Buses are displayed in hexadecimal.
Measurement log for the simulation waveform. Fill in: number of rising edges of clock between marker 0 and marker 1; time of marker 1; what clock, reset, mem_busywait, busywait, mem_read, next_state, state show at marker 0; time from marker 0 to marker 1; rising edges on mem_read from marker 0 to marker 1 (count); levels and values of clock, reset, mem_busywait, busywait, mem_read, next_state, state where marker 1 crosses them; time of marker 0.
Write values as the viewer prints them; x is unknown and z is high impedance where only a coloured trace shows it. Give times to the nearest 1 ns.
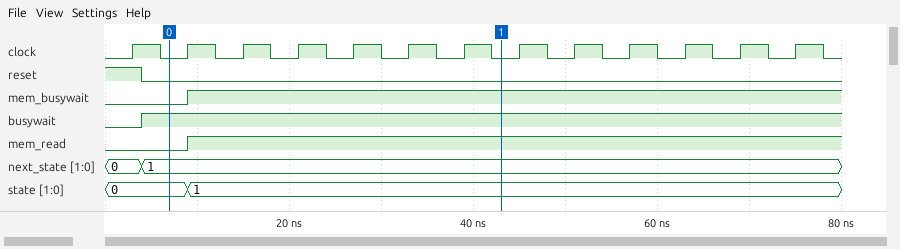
6
43 ns
clock=0, reset=0, mem_busywait=0, busywait=1, mem_read=0, next_state=1, state=0
36 ns
1
clock=0, reset=0, mem_busywait=1, busywait=1, mem_read=1, next_state=1, state=1
7 ns
